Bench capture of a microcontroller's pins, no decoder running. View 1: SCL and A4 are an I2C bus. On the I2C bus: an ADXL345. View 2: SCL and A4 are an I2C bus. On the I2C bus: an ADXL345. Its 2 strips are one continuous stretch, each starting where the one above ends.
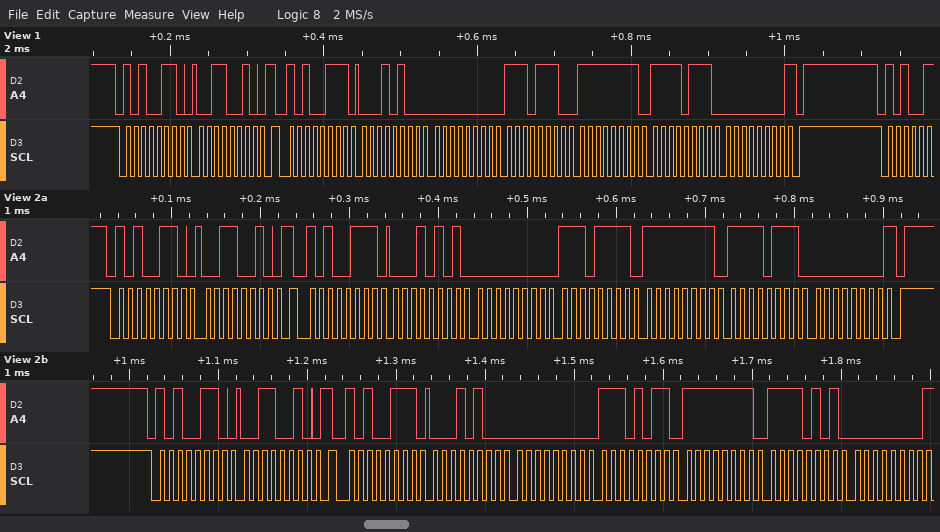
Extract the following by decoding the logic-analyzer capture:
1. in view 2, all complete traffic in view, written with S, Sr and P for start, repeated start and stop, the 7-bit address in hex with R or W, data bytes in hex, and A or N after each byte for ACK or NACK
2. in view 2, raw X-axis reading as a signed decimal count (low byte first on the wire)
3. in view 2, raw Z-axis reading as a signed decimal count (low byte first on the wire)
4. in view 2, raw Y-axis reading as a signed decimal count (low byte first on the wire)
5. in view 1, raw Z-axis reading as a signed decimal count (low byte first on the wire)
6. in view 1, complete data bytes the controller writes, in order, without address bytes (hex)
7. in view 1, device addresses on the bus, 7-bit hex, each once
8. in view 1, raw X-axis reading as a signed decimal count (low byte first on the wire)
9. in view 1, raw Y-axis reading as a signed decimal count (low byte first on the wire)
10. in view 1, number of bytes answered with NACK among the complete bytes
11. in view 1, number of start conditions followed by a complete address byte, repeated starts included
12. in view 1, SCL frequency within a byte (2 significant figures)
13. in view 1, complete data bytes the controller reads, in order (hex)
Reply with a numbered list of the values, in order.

1. S 53W A 32 A Sr 53R A 15 A 00 A EF A FF A F7 A 00 N P S 53W A 32 A Sr 53R A 14 A 00 A EB A FF A F5 A 00 N
2. 21
3. 247
4. -17
5. 247
6. 32
7. 0x53
8. 20
9. -18
10. 1
11. 2
12. 100 kHz
13. 14 00 EE FF F7 00
